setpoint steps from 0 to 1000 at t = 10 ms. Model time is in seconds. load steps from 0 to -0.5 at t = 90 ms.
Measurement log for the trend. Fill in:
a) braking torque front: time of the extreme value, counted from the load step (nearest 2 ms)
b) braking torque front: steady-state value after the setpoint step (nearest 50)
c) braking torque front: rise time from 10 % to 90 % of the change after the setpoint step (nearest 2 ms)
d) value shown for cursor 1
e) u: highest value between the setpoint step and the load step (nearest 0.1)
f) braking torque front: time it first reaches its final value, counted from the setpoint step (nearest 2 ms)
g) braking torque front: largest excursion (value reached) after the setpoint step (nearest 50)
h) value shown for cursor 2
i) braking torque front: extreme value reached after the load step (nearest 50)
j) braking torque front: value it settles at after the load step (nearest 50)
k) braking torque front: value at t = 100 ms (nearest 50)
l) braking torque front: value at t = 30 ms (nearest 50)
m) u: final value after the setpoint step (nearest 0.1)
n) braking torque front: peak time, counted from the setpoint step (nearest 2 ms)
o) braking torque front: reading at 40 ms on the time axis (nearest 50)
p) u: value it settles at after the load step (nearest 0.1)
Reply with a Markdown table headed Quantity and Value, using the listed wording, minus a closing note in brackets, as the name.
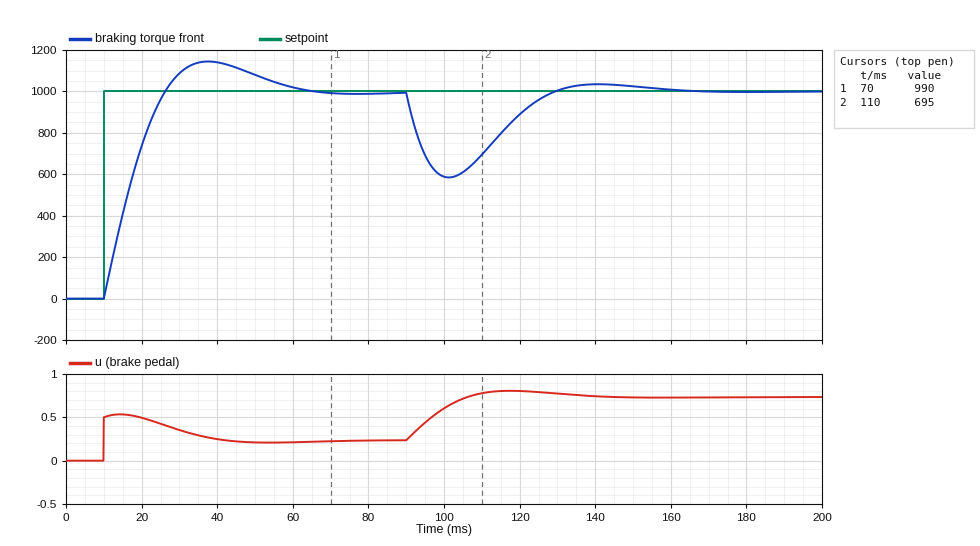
| Quantity | Value |
|---|---|
| braking torque front: time of the extreme value, counted from the load step | 12 ms |
| braking torque front: steady-state value after the setpoint step | 1000 |
| braking torque front: rise time from 10 % to 90 % of the change after the setpoint step | 12 ms |
| value shown for cursor 1 | 990 |
| u: highest value between the setpoint step and the load step | 0.5 |
| braking torque front: time it first reaches its final value, counted from the setpoint step | 16 ms |
| braking torque front: largest excursion (value reached) after the setpoint step | 1150 |
| value shown for cursor 2 | 695 |
| braking torque front: extreme value reached after the load step | 600 |
| braking torque front: value it settles at after the load step | 1000 |
| braking torque front: value at t = 100 ms | 600 |
| braking torque front: value at t = 30 ms | 1100 |
| u: final value after the setpoint step | 0.2 |
| braking torque front: peak time, counted from the setpoint step | 28 ms |
| braking torque front: reading at 40 ms on the time axis | 1150 |
| u: value it settles at after the load step | 0.7 |
